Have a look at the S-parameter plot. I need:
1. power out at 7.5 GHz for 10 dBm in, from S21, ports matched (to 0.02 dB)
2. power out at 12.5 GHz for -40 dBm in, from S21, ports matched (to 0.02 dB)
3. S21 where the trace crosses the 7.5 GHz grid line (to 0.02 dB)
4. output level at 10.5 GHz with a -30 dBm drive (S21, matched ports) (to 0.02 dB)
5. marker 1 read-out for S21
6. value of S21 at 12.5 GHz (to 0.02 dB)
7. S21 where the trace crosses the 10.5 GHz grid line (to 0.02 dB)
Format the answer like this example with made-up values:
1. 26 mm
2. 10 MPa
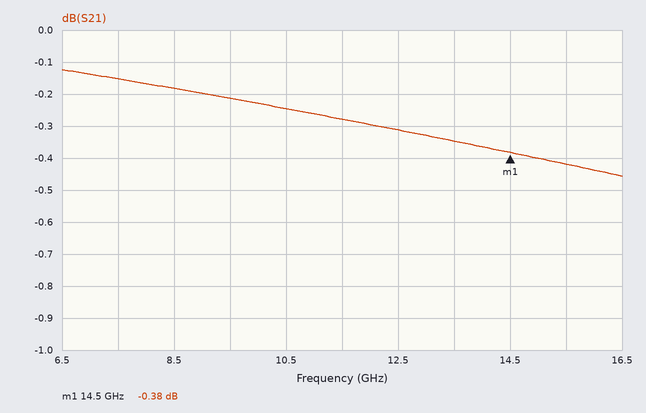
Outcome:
1. 9.84 dBm
2. -40.32 dBm
3. -0.16 dB
4. -30.24 dBm
5. -0.38 dB
6. -0.32 dB
7. -0.24 dB
